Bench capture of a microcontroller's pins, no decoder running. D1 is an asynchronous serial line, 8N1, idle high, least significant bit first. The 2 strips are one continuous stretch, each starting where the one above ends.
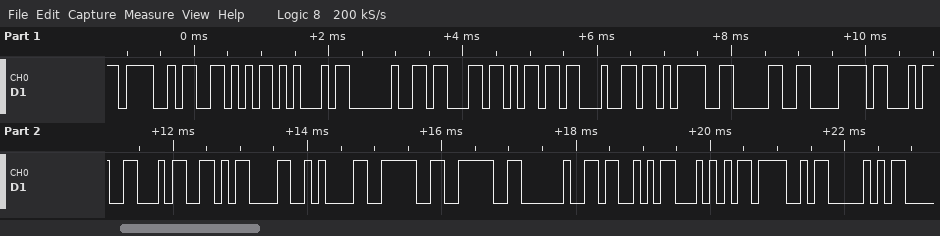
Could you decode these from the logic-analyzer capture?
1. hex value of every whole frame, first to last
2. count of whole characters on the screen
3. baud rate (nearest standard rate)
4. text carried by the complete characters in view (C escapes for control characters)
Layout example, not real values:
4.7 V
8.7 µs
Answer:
4F 56 45 20 63 6D 64 3D 30 78 34 34 0D 0A 3E 3E 20 53 54 4F 50
21
9600 baud
"OVE cmd=0x44\r\n>> STOP"
